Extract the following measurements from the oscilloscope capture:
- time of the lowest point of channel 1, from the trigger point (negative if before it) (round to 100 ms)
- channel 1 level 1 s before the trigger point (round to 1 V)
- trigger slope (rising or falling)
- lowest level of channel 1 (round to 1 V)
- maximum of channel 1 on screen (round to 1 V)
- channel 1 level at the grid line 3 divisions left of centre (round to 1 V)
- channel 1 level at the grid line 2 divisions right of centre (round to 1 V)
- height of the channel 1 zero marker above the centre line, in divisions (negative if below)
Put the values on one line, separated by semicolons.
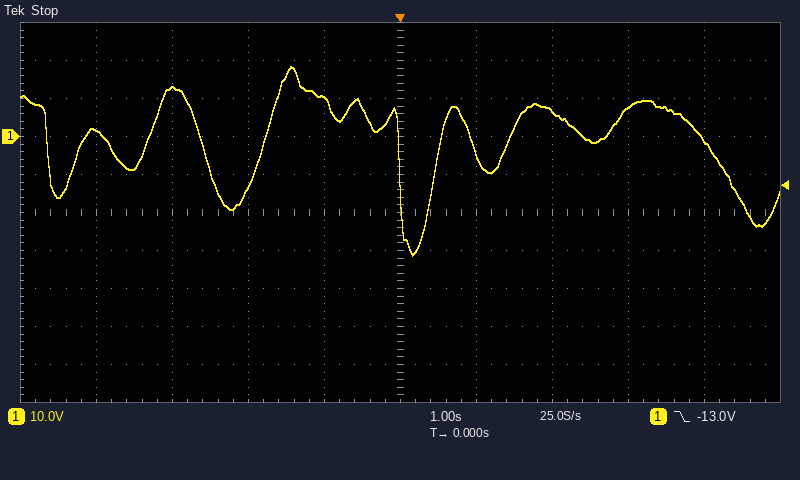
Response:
+200 ms; 10 V; falling; -31 V; 18 V; 13 V; 7 V; +2.0 div
